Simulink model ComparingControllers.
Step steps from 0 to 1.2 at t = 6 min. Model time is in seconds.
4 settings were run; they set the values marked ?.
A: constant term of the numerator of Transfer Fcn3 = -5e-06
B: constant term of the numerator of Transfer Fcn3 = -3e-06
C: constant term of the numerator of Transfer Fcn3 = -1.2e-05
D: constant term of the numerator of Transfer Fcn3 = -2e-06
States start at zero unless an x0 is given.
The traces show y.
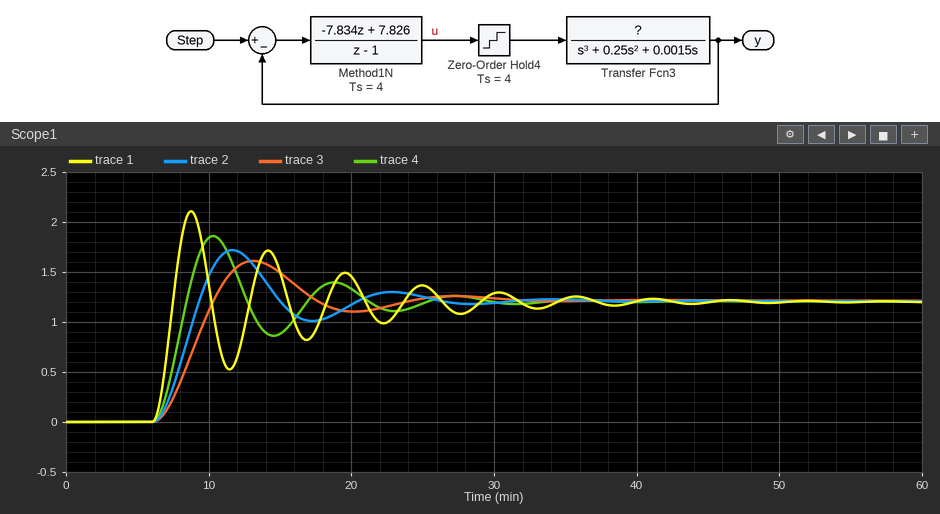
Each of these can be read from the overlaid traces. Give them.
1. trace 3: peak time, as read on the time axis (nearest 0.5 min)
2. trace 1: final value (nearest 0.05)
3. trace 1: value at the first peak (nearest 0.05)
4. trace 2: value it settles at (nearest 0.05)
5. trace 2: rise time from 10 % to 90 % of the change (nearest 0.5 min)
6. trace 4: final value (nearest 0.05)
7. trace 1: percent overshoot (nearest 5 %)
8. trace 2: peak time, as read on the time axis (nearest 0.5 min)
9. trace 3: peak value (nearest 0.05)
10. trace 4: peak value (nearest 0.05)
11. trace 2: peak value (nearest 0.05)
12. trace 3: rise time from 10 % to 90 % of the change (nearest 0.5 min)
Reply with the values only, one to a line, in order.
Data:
13.0 min
1.20
2.10
1.20
2.0 min
1.20
75 %
11.5 min
1.60
1.85
1.70
3.0 min
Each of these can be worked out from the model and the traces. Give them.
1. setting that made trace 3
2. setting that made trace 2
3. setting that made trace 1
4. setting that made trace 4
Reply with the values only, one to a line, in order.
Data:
D
B
C
A
